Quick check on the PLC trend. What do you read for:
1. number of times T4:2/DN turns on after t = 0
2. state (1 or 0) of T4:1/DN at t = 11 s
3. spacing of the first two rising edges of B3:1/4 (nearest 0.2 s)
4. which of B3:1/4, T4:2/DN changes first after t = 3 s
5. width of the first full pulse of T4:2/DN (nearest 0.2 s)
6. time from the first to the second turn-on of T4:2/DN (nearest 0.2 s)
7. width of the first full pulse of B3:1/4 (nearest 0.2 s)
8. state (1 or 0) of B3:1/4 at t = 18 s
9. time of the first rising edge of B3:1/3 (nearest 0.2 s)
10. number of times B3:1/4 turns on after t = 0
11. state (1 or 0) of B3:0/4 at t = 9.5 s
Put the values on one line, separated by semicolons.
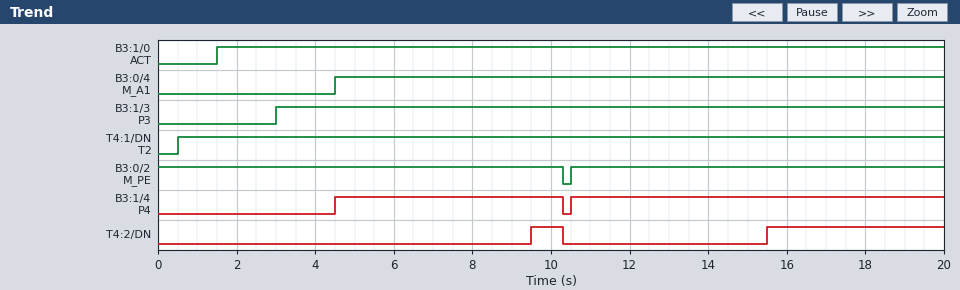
2; 1; 6.0 s; B3:1/4; 0.8 s; 6.0 s; 5.8 s; 1; 3.0 s; 2; 1
